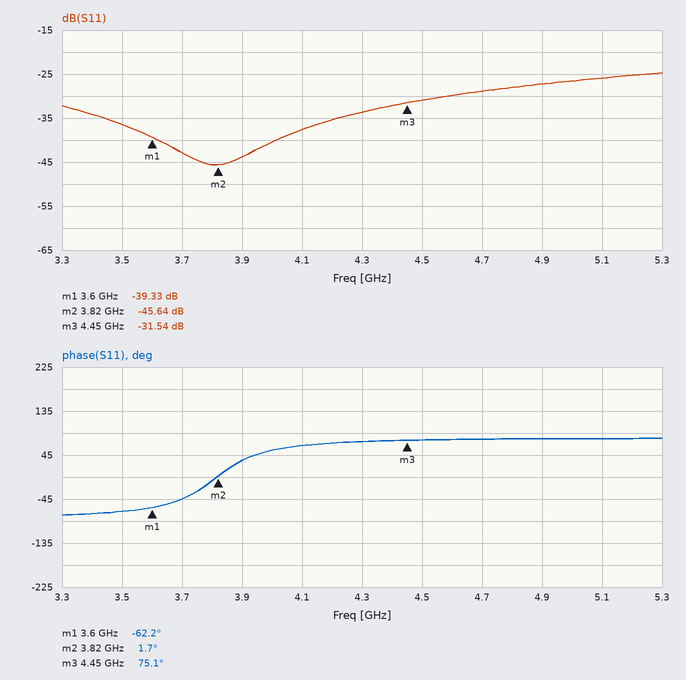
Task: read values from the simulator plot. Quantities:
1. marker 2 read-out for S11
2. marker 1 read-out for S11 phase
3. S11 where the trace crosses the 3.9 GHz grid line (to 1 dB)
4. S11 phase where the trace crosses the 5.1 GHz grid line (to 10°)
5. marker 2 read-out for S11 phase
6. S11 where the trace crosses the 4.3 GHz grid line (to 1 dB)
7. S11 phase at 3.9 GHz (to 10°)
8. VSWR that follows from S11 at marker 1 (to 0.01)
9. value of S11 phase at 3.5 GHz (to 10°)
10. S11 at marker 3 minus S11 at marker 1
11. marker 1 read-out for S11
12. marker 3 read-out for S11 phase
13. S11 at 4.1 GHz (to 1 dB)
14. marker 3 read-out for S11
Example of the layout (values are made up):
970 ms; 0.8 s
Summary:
-45.64 dB; -62.2°; -44 dB; 80°; 1.7°; -34 dB; 30°; 1.02; -70°; 7.79 dB; -39.33 dB; 75.1°; -38 dB; -31.54 dB
